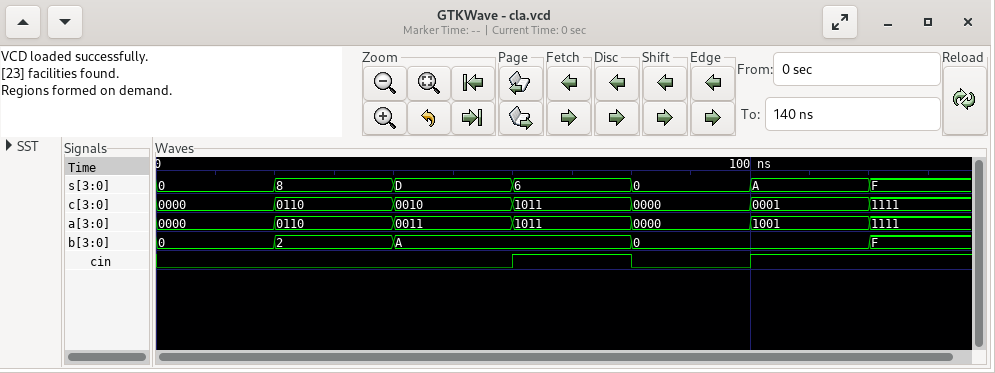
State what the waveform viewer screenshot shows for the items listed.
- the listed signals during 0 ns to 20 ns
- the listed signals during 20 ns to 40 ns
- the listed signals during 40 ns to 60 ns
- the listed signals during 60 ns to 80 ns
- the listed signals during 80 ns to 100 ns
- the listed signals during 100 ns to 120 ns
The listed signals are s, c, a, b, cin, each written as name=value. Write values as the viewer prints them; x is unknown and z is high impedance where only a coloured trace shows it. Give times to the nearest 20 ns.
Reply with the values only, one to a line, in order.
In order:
s=0, c=0000, a=0000, b=0, cin=0
s=8, c=0110, a=0110, b=2, cin=0
s=D, c=0010, a=0011, b=A, cin=0
s=6, c=1011, a=1011, b=A, cin=1
s=0, c=0000, a=0000, b=0, cin=0
s=A, c=0001, a=1001, b=0, cin=1
